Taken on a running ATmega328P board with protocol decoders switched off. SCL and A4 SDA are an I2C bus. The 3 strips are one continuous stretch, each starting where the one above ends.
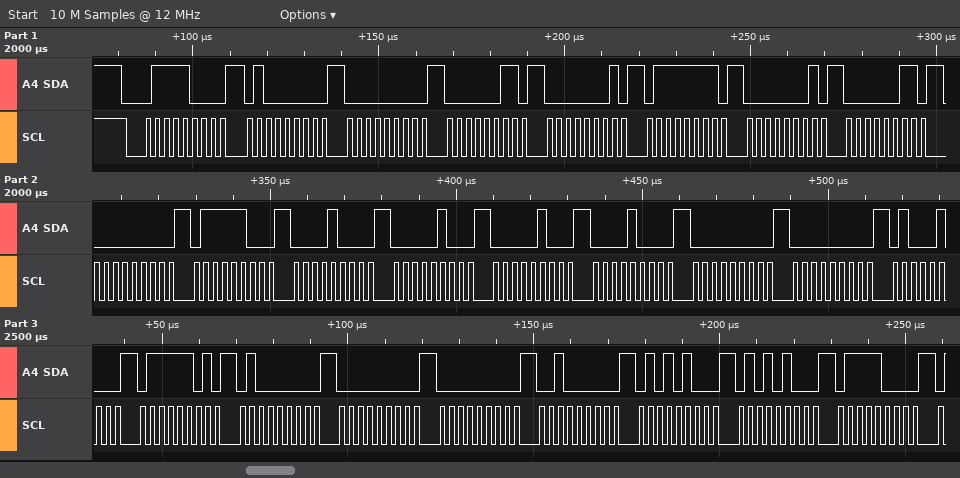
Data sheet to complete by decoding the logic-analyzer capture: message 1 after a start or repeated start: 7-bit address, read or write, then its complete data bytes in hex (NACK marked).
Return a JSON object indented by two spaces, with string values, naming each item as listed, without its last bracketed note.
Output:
{
  "message 1 after a start or repeated start: 7-bit address, read or write, then its complete data bytes in hex": "0x3C write: 40 00 03 01 7F 01 03 00 7C 08 04 04 08 00 00 44 7D 40 00 00 20 54 54 78"
}
